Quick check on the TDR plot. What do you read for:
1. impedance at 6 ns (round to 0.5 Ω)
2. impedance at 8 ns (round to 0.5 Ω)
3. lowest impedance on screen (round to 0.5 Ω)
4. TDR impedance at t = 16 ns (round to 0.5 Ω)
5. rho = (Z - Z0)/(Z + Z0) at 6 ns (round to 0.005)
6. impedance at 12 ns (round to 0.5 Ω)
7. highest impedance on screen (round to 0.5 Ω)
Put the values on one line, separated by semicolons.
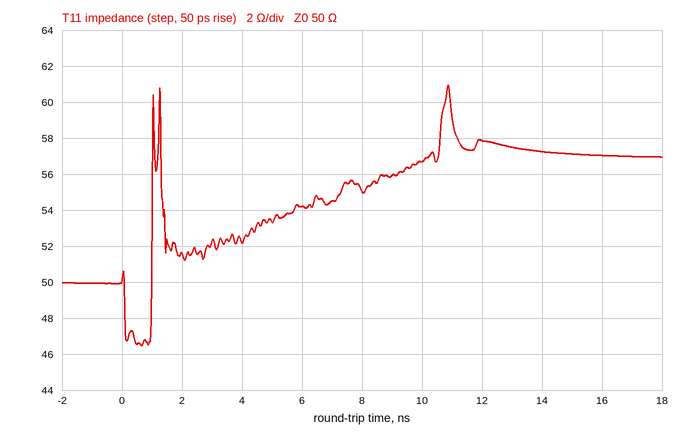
54.0 Ω; 55.0 Ω; 46.5 Ω; 57.0 Ω; +0.040; 58.0 Ω; 61.0 Ω
